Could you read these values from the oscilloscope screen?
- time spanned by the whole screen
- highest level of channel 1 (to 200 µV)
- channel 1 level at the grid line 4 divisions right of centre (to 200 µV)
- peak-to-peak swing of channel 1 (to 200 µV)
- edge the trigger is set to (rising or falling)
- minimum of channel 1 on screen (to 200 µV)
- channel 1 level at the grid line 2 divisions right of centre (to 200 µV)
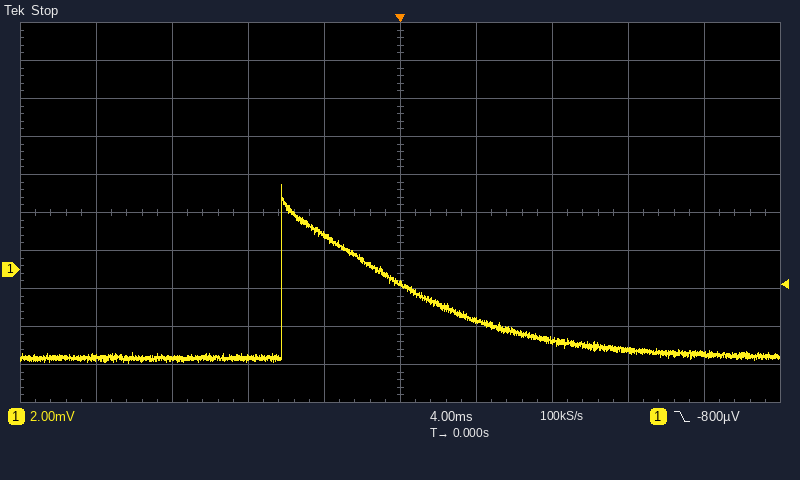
40 ms
4.4 mV
-4.4 mV
9.4 mV
falling
-5.0 mV
-3.8 mV
